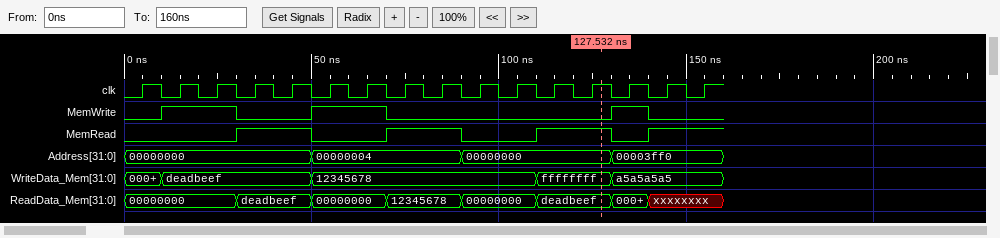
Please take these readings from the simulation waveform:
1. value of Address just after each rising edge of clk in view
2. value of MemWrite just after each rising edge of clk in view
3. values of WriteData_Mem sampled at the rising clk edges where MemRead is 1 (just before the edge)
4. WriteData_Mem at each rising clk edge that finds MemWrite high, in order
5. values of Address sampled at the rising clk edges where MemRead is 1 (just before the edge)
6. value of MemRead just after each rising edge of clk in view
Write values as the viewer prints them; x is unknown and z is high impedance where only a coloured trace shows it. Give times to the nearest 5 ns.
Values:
00000000, 00000000, 00000000, 00000000, 00000000, 00000004, 00000004, 00000004, 00000004, 00000000, 00000000, 00000000, 00000000, 00003ff0, 00003ff0, 00003ff0
0 1 1 0 0 1 1 0 0 0 0 0 0 1 0 0
deadbeef, deadbeef, 12345678, 12345678, ffffffff, ffffffff, a5a5a5a5, a5a5a5a5
deadbeef, deadbeef, 12345678, 12345678, a5a5a5a5
00000000, 00000000, 00000004, 00000004, 00000000, 00000000, 00003ff0, 00003ff0
0 0 0 1 1 0 0 1 1 0 0 1 1 0 1 1
